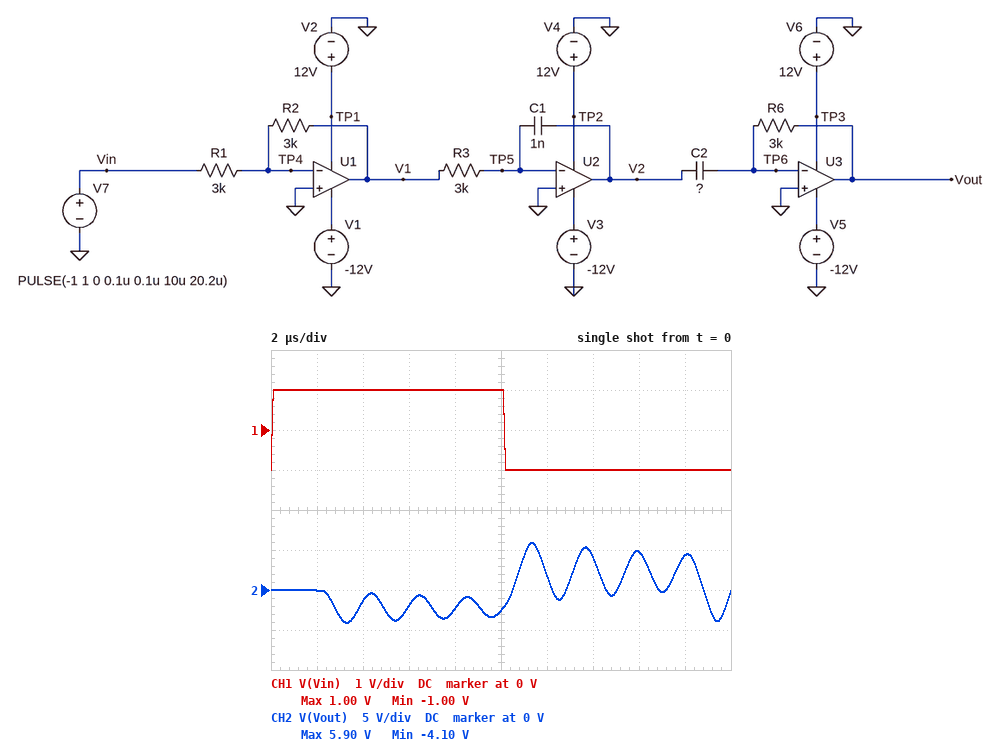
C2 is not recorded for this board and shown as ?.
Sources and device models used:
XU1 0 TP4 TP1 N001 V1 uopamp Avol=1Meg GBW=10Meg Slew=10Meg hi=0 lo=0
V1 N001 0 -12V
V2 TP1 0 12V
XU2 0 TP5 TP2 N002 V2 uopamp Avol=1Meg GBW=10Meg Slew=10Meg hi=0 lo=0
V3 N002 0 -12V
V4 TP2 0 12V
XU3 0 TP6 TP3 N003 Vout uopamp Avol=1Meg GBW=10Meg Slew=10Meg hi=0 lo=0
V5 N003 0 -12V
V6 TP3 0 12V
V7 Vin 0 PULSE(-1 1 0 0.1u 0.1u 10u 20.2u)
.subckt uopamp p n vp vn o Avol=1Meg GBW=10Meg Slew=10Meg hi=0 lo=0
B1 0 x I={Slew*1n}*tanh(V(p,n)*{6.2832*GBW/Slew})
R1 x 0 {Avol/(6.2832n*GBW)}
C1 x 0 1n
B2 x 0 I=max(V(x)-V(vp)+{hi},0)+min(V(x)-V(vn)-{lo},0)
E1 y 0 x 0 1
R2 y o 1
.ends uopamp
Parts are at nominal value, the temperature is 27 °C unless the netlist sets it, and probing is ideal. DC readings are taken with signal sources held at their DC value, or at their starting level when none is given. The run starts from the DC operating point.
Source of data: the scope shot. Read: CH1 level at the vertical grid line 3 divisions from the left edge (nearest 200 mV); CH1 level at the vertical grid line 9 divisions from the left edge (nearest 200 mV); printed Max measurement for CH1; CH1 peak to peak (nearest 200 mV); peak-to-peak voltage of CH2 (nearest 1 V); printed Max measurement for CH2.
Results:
1.0 V
-1.0 V
1.00 V
2.0 V
10 V
5.90 V
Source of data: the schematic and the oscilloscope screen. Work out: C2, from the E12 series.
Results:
2.2 nF
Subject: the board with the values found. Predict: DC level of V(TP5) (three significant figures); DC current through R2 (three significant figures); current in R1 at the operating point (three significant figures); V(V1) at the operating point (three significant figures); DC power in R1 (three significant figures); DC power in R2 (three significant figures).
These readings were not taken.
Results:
1.00 V
333 µA
333 µA
1.00 V
333 µW
333 µW
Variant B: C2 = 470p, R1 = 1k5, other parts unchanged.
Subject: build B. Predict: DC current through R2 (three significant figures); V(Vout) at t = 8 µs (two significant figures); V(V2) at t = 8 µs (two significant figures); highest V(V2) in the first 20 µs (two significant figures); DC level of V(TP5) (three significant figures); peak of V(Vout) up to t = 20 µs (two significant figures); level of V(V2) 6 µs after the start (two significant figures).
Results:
667 µA
-820 mV
-8.2 V
-6.8 V
2.00 V
2.1 V
-9.6 V
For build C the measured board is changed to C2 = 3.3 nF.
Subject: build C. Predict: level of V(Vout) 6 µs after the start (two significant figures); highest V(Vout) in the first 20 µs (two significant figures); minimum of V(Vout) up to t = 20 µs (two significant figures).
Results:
-5.5 V
7.5 V
-6.2 V
